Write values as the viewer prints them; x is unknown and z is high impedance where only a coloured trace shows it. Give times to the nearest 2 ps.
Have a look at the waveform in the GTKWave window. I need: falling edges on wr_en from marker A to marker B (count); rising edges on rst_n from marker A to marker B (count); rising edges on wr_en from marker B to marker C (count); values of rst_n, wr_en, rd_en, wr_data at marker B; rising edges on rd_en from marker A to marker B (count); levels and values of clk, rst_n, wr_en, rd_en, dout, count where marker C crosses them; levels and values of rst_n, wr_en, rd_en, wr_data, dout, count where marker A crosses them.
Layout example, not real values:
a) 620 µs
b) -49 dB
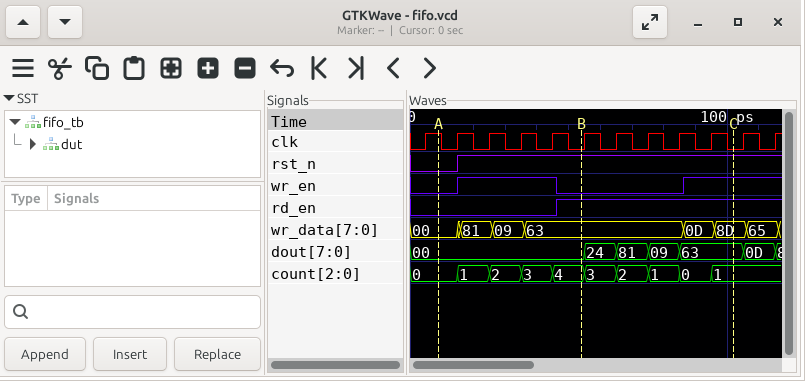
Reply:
a) 1
b) 1
c) 1
d) rst_n=1, wr_en=0, rd_en=1, wr_data=63
e) 1
f) clk=0, rst_n=1, wr_en=1, rd_en=1, dout=63, count=1
g) rst_n=0, wr_en=0, rd_en=0, wr_data=00, dout=00, count=0
